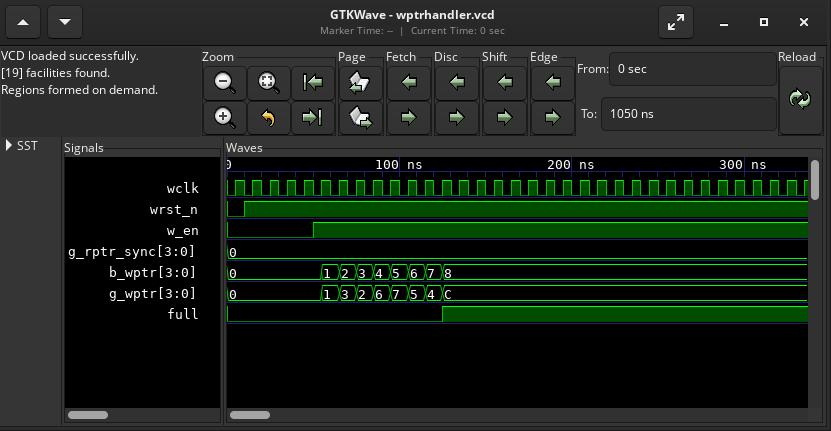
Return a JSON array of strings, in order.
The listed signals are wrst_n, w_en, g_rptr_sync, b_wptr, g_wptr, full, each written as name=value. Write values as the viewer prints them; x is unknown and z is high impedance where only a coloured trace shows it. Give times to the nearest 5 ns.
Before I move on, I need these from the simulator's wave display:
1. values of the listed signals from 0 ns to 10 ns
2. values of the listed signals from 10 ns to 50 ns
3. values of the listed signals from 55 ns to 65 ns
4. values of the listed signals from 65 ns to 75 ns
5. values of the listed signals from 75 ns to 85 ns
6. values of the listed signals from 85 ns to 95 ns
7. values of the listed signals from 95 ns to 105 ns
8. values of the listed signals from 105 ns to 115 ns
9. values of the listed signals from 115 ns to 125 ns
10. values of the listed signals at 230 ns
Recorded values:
["wrst_n=0, w_en=0, g_rptr_sync=0, b_wptr=0, g_wptr=0, full=0", "wrst_n=1, w_en=0, g_rptr_sync=0, b_wptr=0, g_wptr=0, full=0", "wrst_n=1, w_en=1, g_rptr_sync=0, b_wptr=1, g_wptr=1, full=0", "wrst_n=1, w_en=1, g_rptr_sync=0, b_wptr=2, g_wptr=3, full=0", "wrst_n=1, w_en=1, g_rptr_sync=0, b_wptr=3, g_wptr=2, full=0", "wrst_n=1, w_en=1, g_rptr_sync=0, b_wptr=4, g_wptr=6, full=0", "wrst_n=1, w_en=1, g_rptr_sync=0, b_wptr=5, g_wptr=7, full=0", "wrst_n=1, w_en=1, g_rptr_sync=0, b_wptr=6, g_wptr=5, full=0", "wrst_n=1, w_en=1, g_rptr_sync=0, b_wptr=7, g_wptr=4, full=0", "wrst_n=1, w_en=1, g_rptr_sync=0, b_wptr=8, g_wptr=C, full=1"]
